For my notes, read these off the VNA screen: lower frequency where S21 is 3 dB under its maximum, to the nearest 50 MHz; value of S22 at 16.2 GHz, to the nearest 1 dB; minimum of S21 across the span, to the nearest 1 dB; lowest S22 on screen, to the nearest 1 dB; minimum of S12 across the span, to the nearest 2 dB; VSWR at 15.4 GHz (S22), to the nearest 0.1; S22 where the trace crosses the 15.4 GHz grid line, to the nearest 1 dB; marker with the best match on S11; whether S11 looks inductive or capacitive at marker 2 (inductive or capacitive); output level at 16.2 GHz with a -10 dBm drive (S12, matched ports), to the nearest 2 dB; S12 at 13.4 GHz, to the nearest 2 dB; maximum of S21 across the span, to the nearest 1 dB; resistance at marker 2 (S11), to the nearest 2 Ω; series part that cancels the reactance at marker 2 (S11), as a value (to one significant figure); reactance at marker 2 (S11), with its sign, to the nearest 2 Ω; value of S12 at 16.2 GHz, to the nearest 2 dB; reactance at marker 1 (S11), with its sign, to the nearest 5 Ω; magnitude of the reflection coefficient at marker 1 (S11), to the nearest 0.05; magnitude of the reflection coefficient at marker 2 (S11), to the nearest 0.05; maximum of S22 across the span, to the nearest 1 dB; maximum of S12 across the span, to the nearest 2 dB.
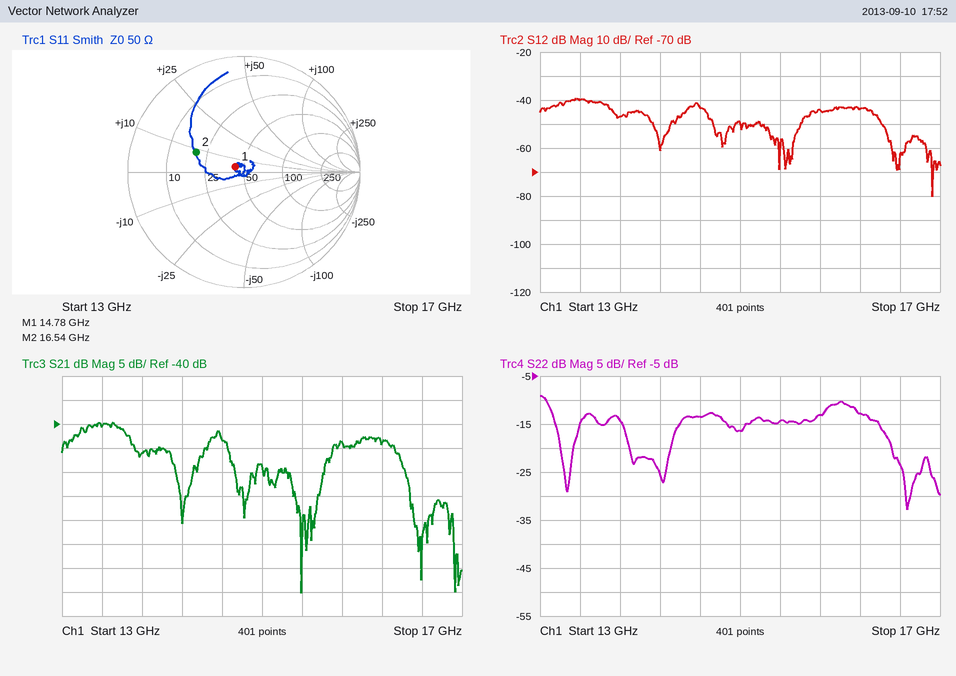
13.10 GHz
-13 dB
-75 dB
-33 dB
-80 dB
1.5
-14 dB
marker 1
inductive
-54 dBm
-40 dB
-40 dB
20 Ω
1 pF
+8 Ω
-44 dB
+5 Ω
0.10
0.45
-9 dB
-40 dB
